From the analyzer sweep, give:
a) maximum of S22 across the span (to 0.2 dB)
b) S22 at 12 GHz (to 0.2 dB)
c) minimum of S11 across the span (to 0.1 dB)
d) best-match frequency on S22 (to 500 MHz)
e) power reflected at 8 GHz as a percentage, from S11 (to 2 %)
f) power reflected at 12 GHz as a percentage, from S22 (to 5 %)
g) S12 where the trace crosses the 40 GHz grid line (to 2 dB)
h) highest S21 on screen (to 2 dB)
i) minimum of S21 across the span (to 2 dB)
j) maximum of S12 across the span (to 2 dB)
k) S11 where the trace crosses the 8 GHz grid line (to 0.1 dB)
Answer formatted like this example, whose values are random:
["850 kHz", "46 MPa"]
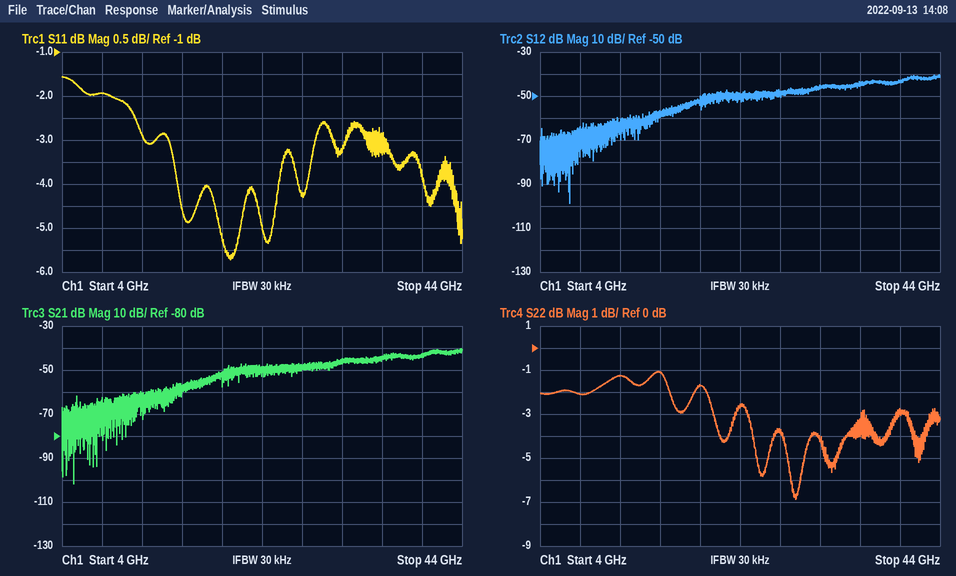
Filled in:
["-1.0 dB", "-1.2 dB", "-5.7 dB", "29.5 GHz", "64 %", "75 %", "-44 dB", "-40 dB", "-102 dB", "-40 dB", "-1.9 dB"]
